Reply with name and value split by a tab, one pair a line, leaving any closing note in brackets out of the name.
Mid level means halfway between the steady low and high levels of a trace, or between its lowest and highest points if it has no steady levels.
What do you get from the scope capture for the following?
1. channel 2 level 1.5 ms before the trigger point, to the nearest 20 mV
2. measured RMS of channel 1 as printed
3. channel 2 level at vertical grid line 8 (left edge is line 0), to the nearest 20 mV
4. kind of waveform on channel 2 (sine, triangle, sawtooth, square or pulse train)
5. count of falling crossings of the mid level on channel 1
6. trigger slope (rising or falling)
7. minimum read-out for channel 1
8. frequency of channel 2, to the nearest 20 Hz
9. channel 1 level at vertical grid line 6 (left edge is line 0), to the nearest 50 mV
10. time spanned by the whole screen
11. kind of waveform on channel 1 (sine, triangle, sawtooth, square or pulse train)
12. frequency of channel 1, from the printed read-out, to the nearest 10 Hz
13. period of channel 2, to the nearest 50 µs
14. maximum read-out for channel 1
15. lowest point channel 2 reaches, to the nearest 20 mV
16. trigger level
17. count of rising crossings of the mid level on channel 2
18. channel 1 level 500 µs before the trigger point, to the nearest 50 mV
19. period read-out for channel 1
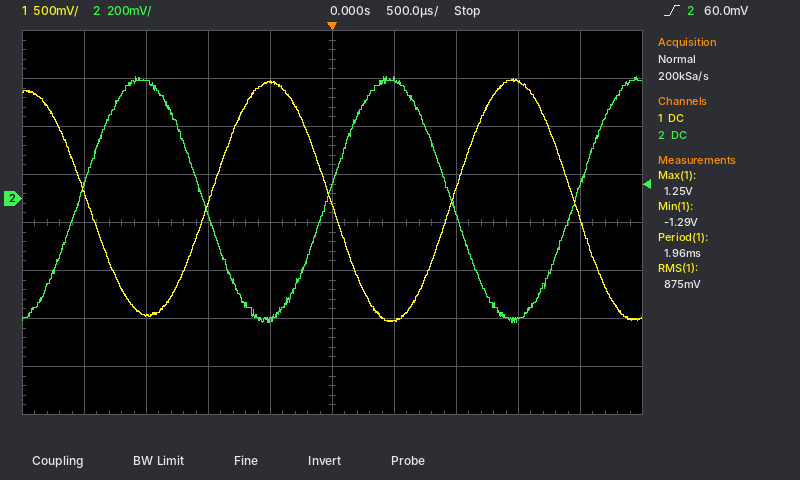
channel 2 level 1.5 ms before the trigger point, to the nearest 20 mV	500 mV
measured RMS of channel 1 as printed	875 mV
channel 2 level at vertical grid line 8 (left edge is line 0), to the nearest 20 mV	-500 mV
kind of waveform on channel 2	sine
count of falling crossings of the mid level on channel 1	3
trigger slope	rising
minimum read-out for channel 1	-1.29 V
frequency of channel 2, to the nearest 20 Hz	500 Hz
channel 1 level at vertical grid line 6 (left edge is line 0), to the nearest 50 mV	-1.25 V
time spanned by the whole screen	5 ms
kind of waveform on channel 1	sine
frequency of channel 1, from the printed read-out, to the nearest 10 Hz	510 Hz
period of channel 2, to the nearest 50 µs	2.00 ms
maximum read-out for channel 1	1.25 V
lowest point channel 2 reaches, to the nearest 20 mV	-520 mV
trigger level	60.0 mV
count of rising crossings of the mid level on channel 2	3
channel 1 level 500 µs before the trigger point, to the nearest 50 mV	1.20 V
period read-out for channel 1	1.96 ms
